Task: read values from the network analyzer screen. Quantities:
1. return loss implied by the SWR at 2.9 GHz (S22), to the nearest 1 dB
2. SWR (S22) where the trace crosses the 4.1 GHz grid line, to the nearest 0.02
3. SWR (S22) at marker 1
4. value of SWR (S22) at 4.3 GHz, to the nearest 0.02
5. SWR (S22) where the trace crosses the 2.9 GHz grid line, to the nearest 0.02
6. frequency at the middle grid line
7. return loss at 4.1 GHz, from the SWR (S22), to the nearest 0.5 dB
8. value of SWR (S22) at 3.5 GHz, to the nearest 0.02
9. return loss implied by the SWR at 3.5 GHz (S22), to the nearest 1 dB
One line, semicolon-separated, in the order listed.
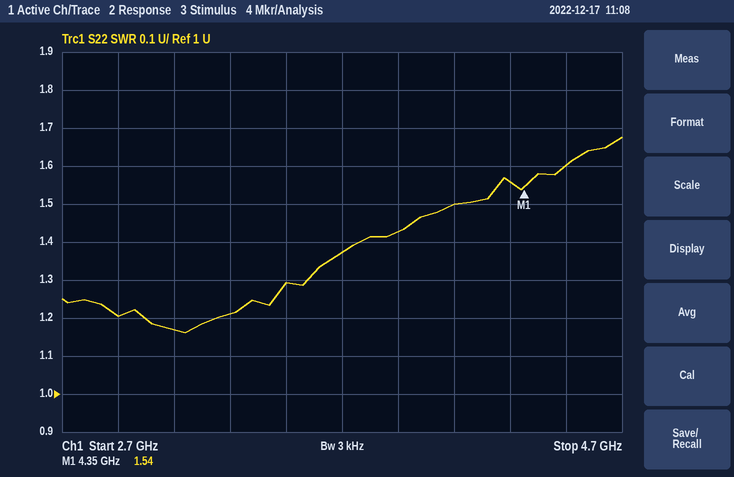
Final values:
21 dB; 1.50; 1.54; 1.56; 1.20; 3.7 GHz; 14.0 dB; 1.30; 18 dB
